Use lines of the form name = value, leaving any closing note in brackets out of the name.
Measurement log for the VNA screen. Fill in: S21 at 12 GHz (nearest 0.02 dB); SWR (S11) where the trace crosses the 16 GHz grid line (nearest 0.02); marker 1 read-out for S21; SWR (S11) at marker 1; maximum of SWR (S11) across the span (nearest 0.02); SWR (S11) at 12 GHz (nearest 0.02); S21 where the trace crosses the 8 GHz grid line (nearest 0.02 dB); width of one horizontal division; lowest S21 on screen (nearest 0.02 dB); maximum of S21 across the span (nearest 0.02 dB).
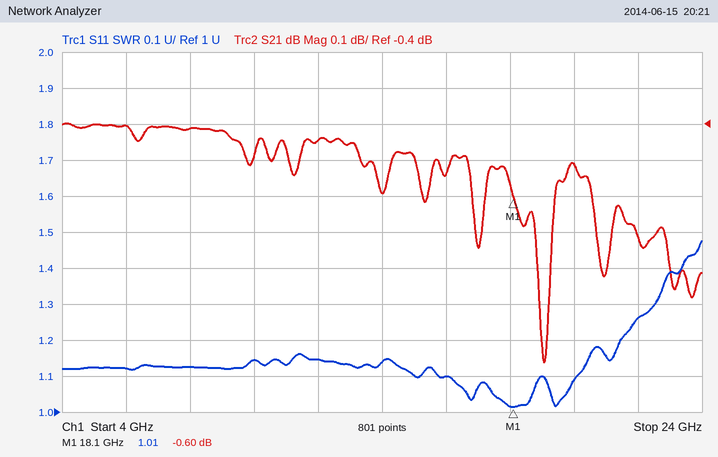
S21 at 12 GHz = -0.44 dB
SWR (S11) where the trace crosses the 16 GHz grid line = 1.10
marker 1 read-out for S21 = -0.60 dB
SWR (S11) at marker 1 = 1.01
maximum of SWR (S11) across the span = 1.48
SWR (S11) at 12 GHz = 1.14
S21 where the trace crosses the 8 GHz grid line = -0.42 dB
width of one horizontal division = 2 GHz
lowest S21 on screen = -1.06 dB
maximum of S21 across the span = -0.40 dB
